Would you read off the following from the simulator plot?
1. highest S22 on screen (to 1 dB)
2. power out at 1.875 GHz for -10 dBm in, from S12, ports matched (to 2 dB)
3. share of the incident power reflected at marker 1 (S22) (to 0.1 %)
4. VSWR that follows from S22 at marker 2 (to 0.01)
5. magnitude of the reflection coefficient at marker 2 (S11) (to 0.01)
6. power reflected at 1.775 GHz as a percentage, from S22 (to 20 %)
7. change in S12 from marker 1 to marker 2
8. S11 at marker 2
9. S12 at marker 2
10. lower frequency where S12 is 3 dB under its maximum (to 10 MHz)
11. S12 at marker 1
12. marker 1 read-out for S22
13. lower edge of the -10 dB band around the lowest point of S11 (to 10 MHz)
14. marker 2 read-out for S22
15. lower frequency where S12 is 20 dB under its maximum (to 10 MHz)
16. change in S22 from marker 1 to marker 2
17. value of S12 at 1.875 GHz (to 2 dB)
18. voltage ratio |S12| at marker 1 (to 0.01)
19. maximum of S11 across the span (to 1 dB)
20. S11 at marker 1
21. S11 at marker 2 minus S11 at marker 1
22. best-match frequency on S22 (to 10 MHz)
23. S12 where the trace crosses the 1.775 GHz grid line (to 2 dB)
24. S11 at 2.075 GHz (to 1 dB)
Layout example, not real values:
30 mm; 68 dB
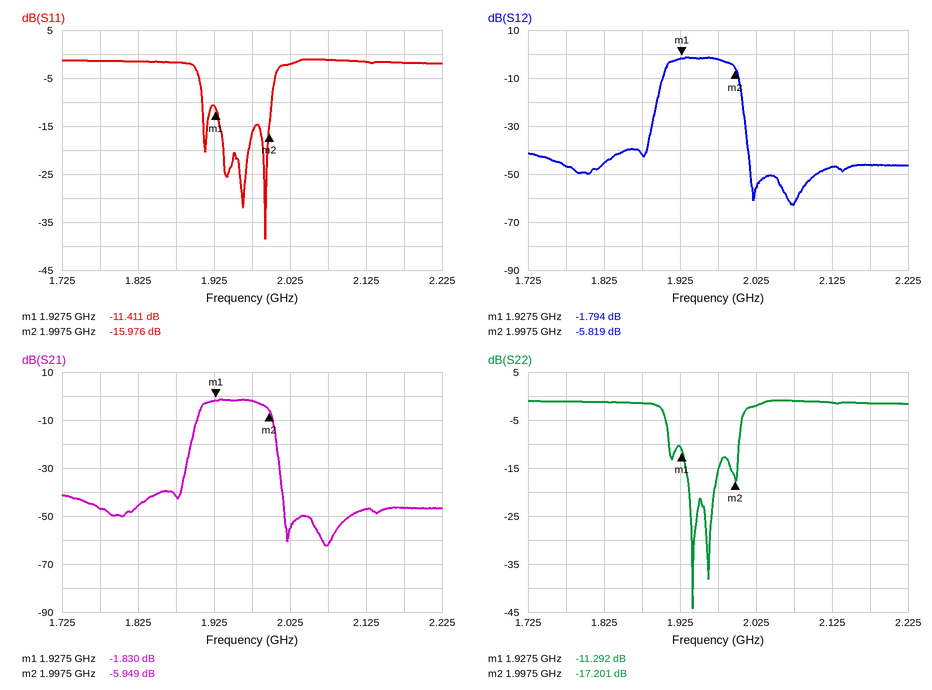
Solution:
-1 dB; -52 dBm; 7.4 %; 1.32; 0.16; 80 %; -4.025 dB; -15.976 dB; -5.819 dB; 1.91 GHz; -1.794 dB; -11.292 dB; 1.91 GHz; -17.201 dB; 1.89 GHz; -5.909 dB; -42 dB; 0.81; -1 dB; -11.411 dB; -4.565 dB; 1.94 GHz; -46 dB; -1 dB
